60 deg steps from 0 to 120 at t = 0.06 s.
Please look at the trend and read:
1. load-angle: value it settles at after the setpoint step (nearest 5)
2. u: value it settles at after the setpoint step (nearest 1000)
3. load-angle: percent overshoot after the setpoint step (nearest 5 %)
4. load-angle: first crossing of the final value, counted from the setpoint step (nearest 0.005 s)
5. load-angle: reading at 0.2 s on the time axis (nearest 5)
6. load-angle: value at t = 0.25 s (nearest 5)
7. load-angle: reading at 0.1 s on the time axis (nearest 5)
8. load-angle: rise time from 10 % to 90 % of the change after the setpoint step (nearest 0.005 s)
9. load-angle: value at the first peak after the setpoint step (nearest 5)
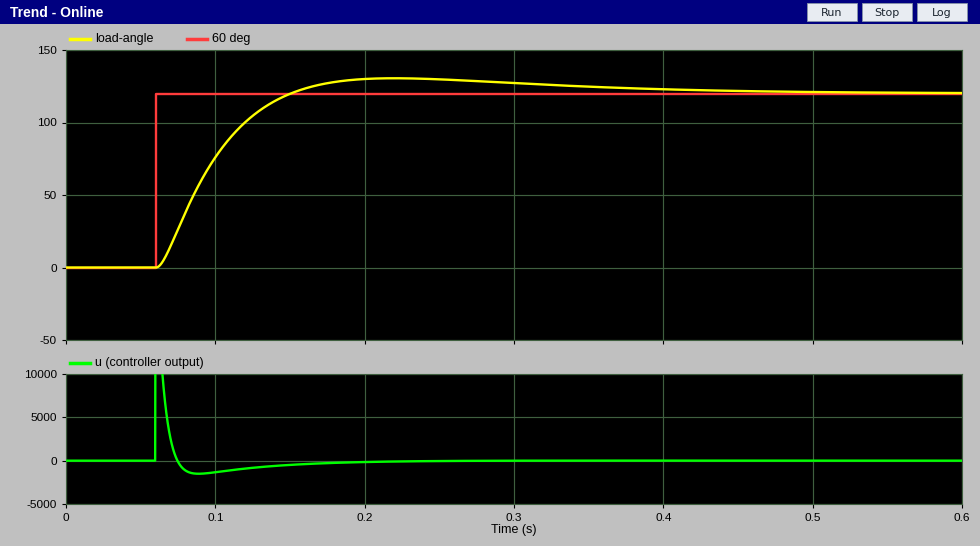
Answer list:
120
0
10 %
0.090 s
130
130
75
0.060 s
130
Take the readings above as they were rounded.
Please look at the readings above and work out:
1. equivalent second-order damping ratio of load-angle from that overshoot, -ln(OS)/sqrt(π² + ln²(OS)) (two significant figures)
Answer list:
0.59
